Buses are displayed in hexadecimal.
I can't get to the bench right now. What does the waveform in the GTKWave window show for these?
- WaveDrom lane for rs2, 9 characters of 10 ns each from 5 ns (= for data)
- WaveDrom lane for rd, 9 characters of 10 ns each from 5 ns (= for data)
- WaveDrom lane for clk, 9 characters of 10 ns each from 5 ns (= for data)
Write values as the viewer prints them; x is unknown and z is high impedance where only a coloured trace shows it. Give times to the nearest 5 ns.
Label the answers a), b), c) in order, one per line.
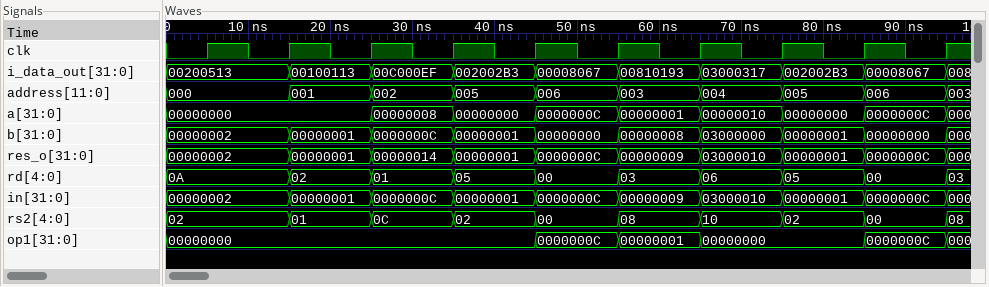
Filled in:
a) {name: 'rs2', wave: '=========', data: '02 01 0C 02 00 08 10 02 00'}
b) {name: 'rd', wave: '=========', data: '0A 02 01 05 00 03 06 05 00'}
c) {name: 'clk', wave: 'p........'}
